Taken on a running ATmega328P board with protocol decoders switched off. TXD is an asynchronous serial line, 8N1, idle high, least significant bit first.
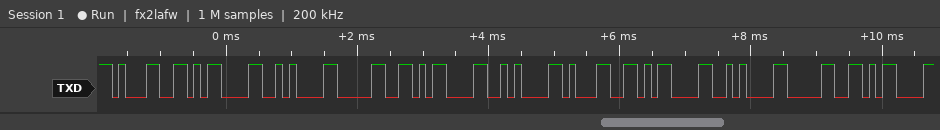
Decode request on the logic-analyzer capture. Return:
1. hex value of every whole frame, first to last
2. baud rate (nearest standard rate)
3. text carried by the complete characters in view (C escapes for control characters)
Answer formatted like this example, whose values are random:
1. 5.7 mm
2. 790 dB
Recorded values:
1. 31 0D 0A 30 0D 0A 31 0D 0A 30 0D
2. 9600 baud
3. "1\r\n0\r\n1\r\n0\r"
